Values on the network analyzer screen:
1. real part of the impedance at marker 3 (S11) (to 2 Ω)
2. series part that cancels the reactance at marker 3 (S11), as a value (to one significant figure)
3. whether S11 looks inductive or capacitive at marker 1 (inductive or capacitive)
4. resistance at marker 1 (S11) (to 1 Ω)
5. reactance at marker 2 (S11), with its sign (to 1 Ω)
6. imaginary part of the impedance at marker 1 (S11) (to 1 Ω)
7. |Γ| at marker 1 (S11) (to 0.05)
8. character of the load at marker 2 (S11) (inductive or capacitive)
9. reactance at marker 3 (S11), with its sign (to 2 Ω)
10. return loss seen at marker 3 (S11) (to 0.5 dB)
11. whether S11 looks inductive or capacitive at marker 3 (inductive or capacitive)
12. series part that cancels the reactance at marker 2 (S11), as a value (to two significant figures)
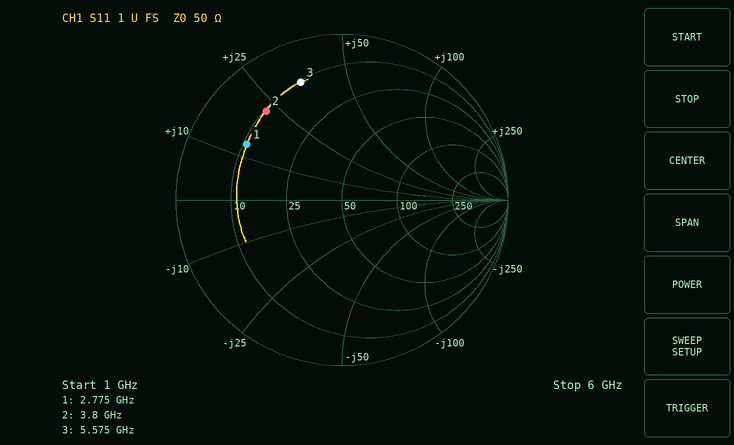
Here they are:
10 Ω
800 fF
inductive
11 Ω
+22 Ω
+13 Ω
0.65
inductive
+34 Ω
2.5 dB
inductive
1.9 pF
